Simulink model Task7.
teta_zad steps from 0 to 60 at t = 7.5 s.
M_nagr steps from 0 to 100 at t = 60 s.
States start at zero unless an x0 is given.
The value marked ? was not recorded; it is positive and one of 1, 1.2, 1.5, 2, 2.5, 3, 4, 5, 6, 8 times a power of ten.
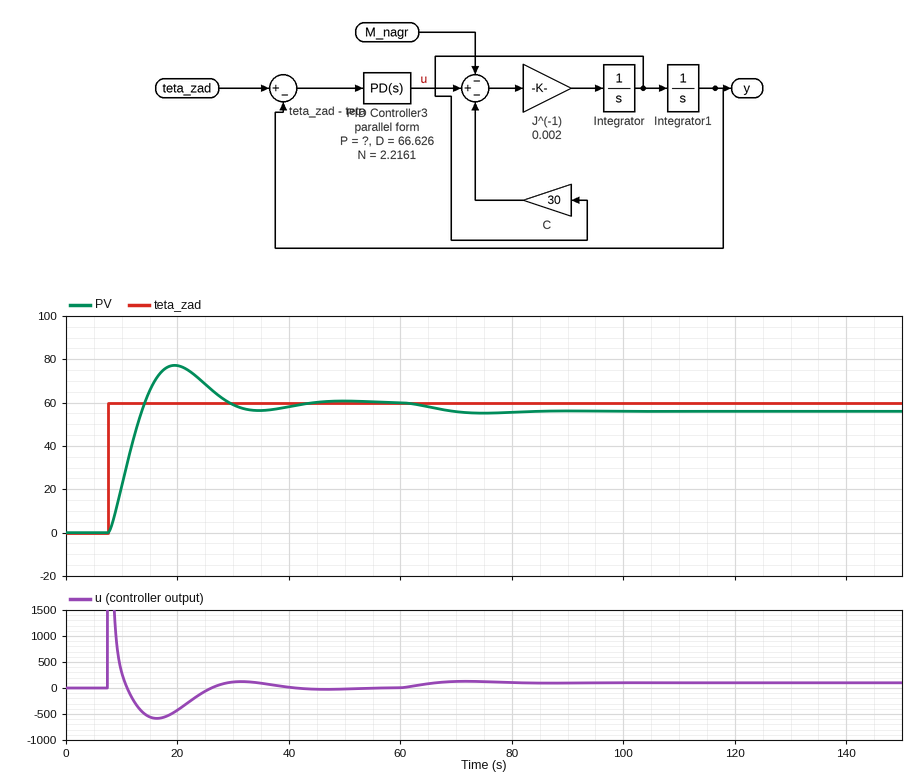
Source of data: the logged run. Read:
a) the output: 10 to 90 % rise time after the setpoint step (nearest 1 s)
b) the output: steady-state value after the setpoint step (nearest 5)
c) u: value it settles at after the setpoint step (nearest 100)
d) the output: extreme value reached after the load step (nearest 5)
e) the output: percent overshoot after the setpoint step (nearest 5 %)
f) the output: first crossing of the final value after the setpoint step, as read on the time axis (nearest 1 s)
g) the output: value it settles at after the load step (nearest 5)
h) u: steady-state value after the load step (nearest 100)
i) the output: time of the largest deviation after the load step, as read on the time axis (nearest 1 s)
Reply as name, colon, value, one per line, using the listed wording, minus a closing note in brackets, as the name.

the output: 10 to 90 % rise time after the setpoint step: 5 s
the output: steady-state value after the setpoint step: 60
u: value it settles at after the setpoint step: 0
the output: extreme value reached after the load step: 55
the output: percent overshoot after the setpoint step: 30 %
the output: first crossing of the final value after the setpoint step, as read on the time axis: 14 s
the output: value it settles at after the load step: 55
u: steady-state value after the load step: 100
the output: time of the largest deviation after the load step, as read on the time axis: 75 s
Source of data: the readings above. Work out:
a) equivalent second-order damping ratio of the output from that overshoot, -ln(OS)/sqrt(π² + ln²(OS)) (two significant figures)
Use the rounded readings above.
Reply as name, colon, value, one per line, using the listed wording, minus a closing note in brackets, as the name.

equivalent second-order damping ratio of the output from that overshoot, -ln(OS)/sqrt(π² + ln²(OS)): 0.36
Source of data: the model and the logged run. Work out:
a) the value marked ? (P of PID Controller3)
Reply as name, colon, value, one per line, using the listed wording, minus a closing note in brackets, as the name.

the value marked ?: 25
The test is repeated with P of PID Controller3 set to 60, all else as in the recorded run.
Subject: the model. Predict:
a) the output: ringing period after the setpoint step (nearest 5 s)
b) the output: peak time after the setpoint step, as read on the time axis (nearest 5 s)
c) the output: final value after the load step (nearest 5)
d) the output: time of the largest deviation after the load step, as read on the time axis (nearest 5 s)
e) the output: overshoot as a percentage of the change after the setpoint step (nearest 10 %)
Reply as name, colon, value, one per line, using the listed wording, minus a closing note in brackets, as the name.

the output: ringing period after the setpoint step: 20 s
the output: peak time after the setpoint step, as read on the time axis: 15 s
the output: final value after the load step: 60
the output: time of the largest deviation after the load step, as read on the time axis: 70 s
the output: overshoot as a percentage of the change after the setpoint step: 50 %
